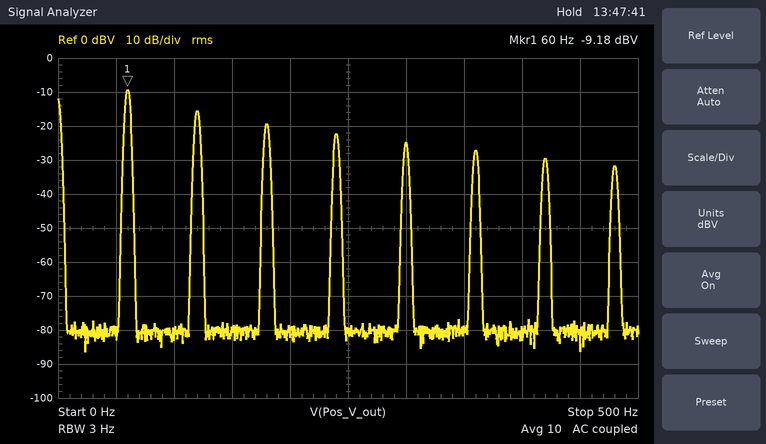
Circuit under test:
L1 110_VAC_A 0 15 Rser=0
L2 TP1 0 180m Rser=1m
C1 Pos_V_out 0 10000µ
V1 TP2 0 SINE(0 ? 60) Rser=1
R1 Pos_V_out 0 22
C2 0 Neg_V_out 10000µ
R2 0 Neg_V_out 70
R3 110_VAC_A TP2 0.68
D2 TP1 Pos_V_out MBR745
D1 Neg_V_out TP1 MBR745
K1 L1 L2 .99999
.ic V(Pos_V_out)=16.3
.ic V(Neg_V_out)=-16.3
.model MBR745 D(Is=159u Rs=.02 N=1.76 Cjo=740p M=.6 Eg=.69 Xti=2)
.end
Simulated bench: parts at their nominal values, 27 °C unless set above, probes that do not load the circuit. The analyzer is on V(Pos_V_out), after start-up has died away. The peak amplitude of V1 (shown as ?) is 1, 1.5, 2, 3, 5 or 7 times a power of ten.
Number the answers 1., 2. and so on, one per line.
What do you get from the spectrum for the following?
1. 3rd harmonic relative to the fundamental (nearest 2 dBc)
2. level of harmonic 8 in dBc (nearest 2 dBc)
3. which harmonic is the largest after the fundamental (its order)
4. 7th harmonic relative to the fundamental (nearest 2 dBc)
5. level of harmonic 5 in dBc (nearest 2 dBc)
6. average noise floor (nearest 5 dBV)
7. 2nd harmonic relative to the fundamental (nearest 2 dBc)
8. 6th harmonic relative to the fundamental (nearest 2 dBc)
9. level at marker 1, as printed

1. -10 dBc
2. -22 dBc
3. 2
4. -20 dBc
5. -16 dBc
6. -80 dBV
7. -6 dBc
8. -18 dBc
9. -9.18 dBV
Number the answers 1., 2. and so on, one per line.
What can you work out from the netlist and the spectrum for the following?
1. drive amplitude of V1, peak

1. 200 V
